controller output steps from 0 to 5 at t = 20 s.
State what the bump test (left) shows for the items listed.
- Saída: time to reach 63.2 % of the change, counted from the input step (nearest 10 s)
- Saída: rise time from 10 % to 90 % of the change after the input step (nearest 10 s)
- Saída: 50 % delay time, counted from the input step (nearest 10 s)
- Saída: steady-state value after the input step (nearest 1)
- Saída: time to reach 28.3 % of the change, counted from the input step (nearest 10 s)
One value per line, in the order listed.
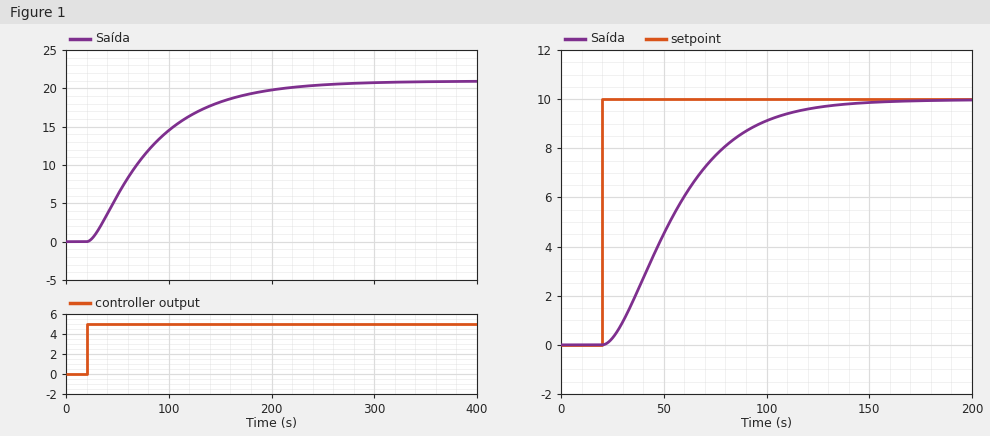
70 s
130 s
50 s
21
30 s
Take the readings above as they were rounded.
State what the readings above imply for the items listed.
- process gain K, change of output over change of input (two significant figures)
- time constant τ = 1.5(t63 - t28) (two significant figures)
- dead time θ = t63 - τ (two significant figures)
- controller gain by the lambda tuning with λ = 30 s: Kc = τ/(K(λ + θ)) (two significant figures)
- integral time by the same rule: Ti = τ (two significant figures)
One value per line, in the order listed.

4.2
60 s
10 s
0.36
60 s
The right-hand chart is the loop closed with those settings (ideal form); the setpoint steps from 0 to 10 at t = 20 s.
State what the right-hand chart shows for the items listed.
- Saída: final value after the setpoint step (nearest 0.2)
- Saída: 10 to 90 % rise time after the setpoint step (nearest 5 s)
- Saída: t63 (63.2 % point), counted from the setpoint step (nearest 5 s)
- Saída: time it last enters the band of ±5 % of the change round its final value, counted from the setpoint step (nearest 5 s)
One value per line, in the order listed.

10.0
65 s
40 s
95 s
